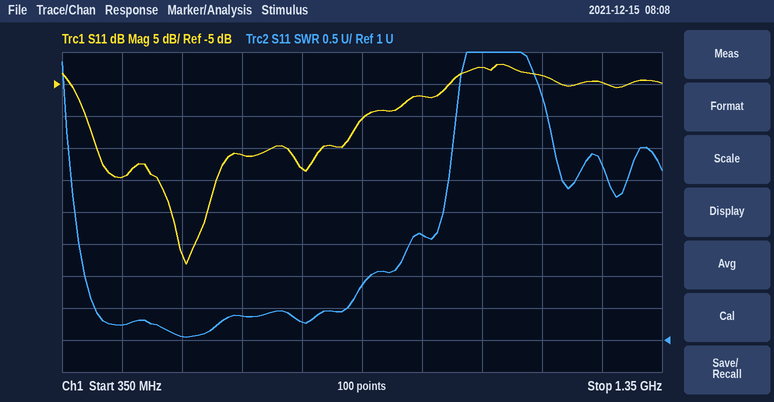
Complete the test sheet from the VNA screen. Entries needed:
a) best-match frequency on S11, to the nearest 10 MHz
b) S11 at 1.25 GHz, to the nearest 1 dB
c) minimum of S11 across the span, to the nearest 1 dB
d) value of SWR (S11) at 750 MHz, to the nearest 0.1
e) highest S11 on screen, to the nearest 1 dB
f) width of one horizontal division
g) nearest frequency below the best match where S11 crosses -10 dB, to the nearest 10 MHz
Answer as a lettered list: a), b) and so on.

a) 560 MHz
b) -5 dB
c) -33 dB
d) 1.3
e) -2 dB
f) 100 MHz
g) 390 MHz
